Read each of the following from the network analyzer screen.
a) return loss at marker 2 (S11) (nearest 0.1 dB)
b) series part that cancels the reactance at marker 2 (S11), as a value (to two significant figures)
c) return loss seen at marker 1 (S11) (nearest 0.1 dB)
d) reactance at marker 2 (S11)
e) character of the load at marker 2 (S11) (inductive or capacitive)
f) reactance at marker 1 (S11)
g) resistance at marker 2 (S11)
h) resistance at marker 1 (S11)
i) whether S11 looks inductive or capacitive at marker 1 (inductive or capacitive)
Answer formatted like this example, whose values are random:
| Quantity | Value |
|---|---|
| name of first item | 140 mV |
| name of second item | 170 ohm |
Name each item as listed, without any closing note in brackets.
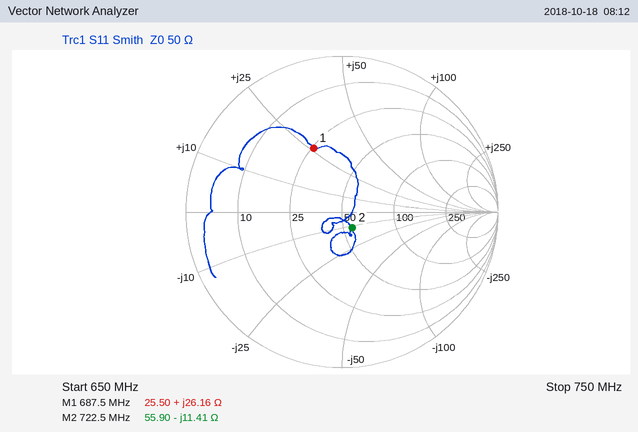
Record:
| Quantity | Value |
|---|---|
| return loss at marker 2 (S11) | 18.4 dB |
| series part that cancels the reactance at marker 2 (S11), as a value | 2.5 nH |
| return loss seen at marker 1 (S11) | 7.0 dB |
| reactance at marker 2 | -11.41 Ω |
| character of the load at marker 2 (S11) | capacitive |
| reactance at marker 1 | +26.16 Ω |
| resistance at marker 2 | 55.90 Ω |
| resistance at marker 1 | 25.50 Ω |
| whether S11 looks inductive or capacitive at marker 1 | inductive |
